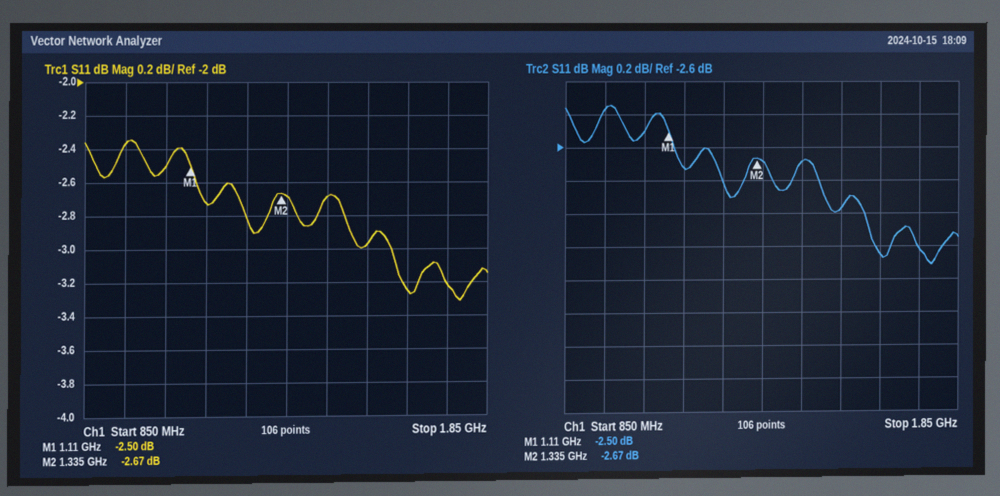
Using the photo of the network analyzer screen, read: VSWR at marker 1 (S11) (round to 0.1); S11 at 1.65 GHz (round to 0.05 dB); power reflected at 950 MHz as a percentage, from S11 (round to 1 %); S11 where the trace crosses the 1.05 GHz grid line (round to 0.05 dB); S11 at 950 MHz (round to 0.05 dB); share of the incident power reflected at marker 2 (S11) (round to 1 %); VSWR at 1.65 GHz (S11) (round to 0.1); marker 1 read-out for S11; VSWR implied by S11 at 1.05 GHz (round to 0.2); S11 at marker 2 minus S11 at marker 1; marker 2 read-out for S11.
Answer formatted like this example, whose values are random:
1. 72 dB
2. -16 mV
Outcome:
1. 7.0
2. -3.25 dB
3. 58 %
4. -2.50 dB
5. -2.35 dB
6. 54 %
7. 5.4
8. -2.50 dB
9. 7.0
10. -0.17 dB
11. -2.67 dB
